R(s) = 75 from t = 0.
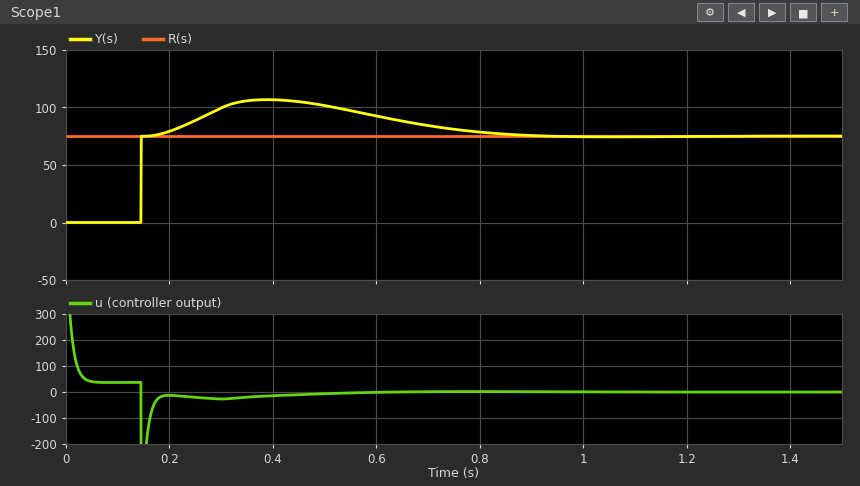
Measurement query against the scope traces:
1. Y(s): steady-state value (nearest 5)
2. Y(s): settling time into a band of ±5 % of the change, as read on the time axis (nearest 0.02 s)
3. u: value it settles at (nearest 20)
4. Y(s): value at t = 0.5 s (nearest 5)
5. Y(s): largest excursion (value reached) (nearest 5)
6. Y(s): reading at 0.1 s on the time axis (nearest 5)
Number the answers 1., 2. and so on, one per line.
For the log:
1. 75
2. 0.80 s
3. 0
4. 100
5. 105
6. 0
